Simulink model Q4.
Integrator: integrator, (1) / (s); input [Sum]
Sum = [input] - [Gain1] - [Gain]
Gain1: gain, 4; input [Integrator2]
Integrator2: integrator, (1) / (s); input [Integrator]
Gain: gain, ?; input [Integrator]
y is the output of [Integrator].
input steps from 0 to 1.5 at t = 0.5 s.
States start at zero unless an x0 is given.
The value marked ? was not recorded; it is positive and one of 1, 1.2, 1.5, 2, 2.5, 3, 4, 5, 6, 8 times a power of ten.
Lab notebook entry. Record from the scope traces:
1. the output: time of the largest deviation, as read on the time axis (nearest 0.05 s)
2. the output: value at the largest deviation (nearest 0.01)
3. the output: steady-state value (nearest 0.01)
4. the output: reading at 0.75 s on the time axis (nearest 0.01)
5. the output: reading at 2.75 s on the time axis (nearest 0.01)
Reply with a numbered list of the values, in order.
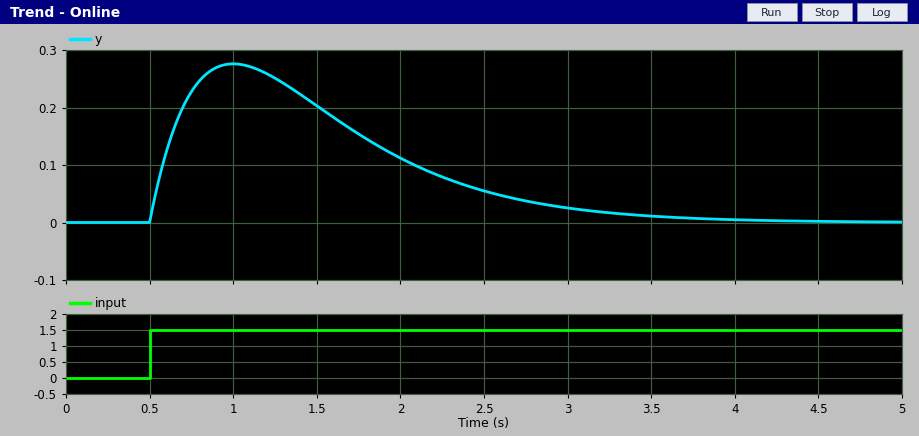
1. 1.00 s
2. 0.28
3. 0.00
4. 0.23
5. 0.04
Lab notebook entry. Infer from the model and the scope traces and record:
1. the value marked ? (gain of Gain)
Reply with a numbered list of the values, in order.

1. 4
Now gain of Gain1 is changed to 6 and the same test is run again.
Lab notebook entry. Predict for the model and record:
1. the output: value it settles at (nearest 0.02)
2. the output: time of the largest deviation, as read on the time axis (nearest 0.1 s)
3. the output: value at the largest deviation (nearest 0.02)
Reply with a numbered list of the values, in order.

1. 0.00
2. 0.9 s
3. 0.26
